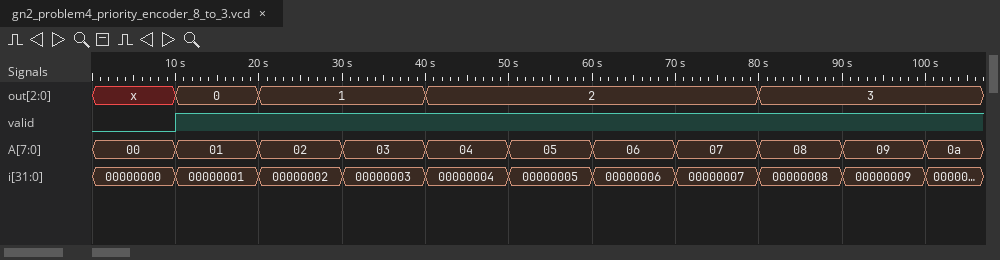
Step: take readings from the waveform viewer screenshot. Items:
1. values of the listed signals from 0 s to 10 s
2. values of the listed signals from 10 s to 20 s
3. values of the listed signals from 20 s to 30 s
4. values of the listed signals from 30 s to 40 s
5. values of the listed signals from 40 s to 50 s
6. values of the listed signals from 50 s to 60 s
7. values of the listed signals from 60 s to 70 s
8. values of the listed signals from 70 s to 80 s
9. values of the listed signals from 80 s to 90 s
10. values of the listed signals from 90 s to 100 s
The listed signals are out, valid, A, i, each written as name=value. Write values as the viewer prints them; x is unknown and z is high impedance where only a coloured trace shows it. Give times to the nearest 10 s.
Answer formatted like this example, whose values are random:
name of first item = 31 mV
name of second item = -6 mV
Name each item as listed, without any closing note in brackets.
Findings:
values of the listed signals from 0 s to 10 s = out=x, valid=0, A=00, i=00000000
values of the listed signals from 10 s to 20 s = out=0, valid=1, A=01, i=00000001
values of the listed signals from 20 s to 30 s = out=1, valid=1, A=02, i=00000002
values of the listed signals from 30 s to 40 s = out=1, valid=1, A=03, i=00000003
values of the listed signals from 40 s to 50 s = out=2, valid=1, A=04, i=00000004
values of the listed signals from 50 s to 60 s = out=2, valid=1, A=05, i=00000005
values of the listed signals from 60 s to 70 s = out=2, valid=1, A=06, i=00000006
values of the listed signals from 70 s to 80 s = out=2, valid=1, A=07, i=00000007
values of the listed signals from 80 s to 90 s = out=3, valid=1, A=08, i=00000008
values of the listed signals from 90 s to 100 s = out=3, valid=1, A=09, i=00000009
